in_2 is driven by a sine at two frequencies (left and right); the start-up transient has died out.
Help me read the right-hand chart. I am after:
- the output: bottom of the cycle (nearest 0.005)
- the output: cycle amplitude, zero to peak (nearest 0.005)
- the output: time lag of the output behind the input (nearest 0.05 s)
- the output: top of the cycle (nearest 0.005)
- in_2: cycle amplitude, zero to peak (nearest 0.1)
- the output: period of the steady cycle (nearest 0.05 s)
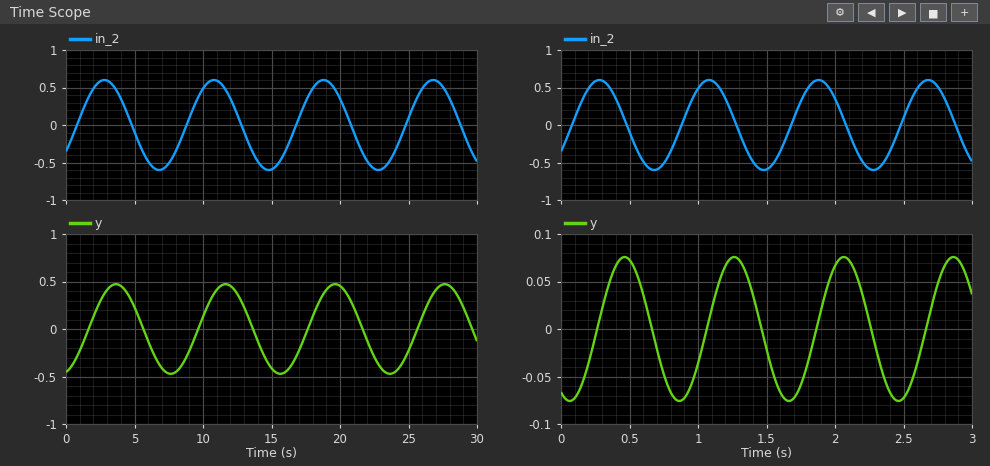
-0.075
0.075
0.20 s
0.075
0.6
0.80 s
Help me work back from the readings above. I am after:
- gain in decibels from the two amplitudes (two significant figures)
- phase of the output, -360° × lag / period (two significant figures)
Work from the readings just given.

-18 dB
-90°
